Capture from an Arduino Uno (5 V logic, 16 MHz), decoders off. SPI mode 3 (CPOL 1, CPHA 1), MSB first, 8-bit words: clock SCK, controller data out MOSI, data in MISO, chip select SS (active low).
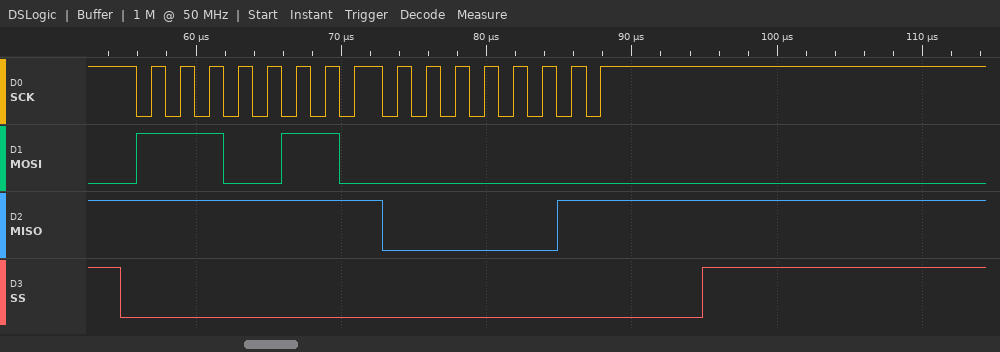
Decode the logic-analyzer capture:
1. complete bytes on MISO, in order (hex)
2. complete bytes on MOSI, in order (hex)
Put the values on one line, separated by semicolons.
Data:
FF 03; E6 00
